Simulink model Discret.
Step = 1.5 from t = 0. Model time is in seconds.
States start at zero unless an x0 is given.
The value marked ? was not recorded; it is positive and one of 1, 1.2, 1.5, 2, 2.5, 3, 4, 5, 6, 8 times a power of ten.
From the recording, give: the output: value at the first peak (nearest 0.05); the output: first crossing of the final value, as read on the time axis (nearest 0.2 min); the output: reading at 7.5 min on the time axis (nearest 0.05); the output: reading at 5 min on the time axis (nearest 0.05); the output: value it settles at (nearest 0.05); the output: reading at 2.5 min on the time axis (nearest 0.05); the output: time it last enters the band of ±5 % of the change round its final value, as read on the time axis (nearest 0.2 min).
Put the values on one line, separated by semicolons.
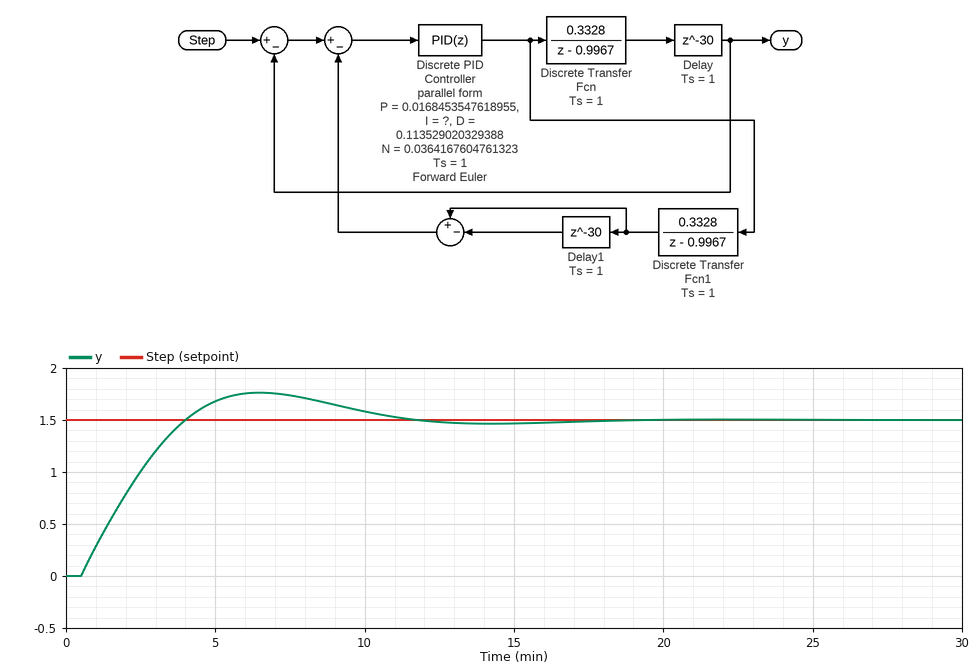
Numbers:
1.75; 4.0 min; 1.75; 1.70; 1.50; 1.00; 10.2 min
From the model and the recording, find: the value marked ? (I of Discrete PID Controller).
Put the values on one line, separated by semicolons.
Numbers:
0.0002
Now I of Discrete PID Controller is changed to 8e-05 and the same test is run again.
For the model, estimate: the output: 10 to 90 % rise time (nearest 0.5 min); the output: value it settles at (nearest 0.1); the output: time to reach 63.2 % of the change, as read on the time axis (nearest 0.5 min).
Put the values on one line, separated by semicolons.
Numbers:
5.0 min; 1.5; 3.0 min
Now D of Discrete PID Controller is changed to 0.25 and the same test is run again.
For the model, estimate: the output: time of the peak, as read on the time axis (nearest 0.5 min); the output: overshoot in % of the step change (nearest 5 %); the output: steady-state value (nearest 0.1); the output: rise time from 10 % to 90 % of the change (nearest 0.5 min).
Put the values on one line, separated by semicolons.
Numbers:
6.5 min; 15 %; 1.5; 3.0 min
